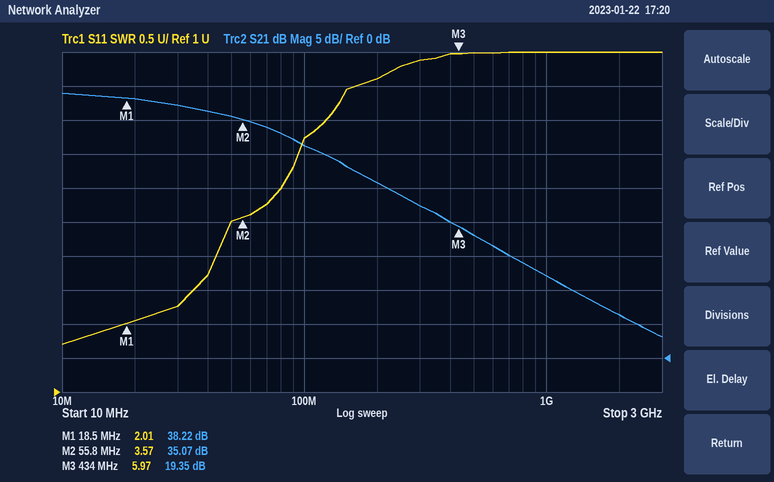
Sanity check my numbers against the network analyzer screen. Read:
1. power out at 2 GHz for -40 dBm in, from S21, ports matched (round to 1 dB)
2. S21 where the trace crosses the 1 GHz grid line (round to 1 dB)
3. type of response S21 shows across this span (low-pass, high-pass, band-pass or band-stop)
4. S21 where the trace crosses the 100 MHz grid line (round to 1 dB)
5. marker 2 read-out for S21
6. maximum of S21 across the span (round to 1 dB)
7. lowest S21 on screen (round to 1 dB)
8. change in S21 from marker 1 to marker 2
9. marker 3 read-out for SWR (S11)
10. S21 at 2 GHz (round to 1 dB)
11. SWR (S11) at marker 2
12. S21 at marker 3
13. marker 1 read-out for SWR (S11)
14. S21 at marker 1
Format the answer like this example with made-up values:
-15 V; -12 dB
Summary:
-34 dBm; 12 dB; low-pass; 31 dB; 35.07 dB; 39 dB; 3 dB; -3.15 dB; 5.97; 6 dB; 3.57; 19.35 dB; 2.01; 38.22 dB
